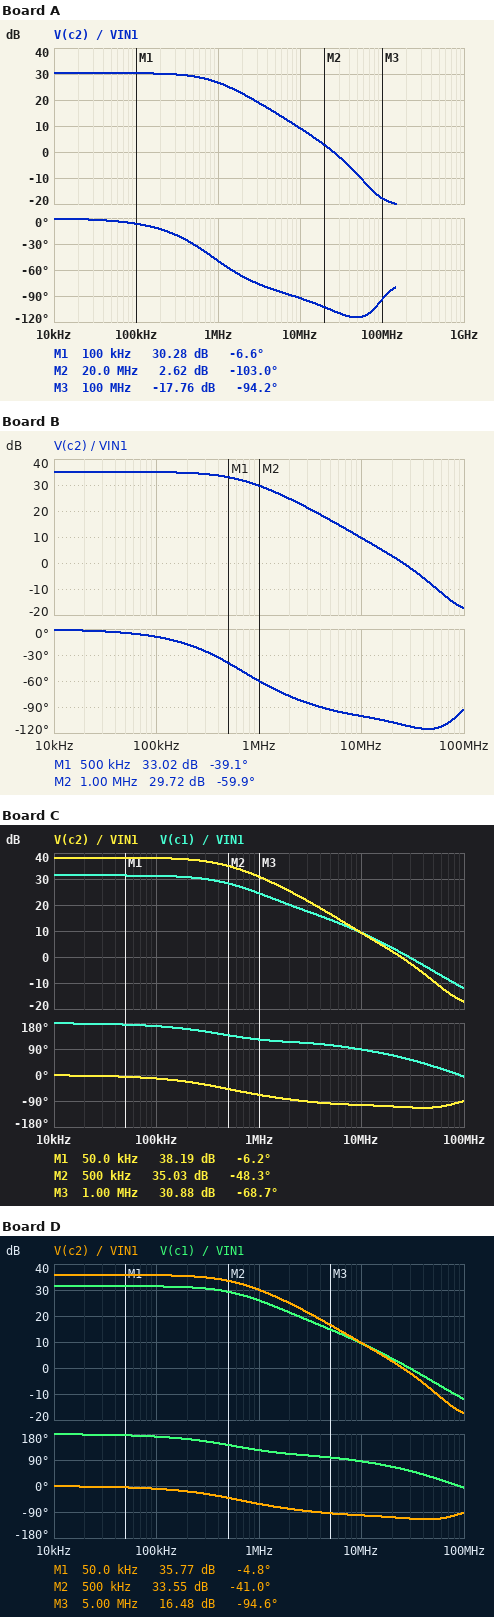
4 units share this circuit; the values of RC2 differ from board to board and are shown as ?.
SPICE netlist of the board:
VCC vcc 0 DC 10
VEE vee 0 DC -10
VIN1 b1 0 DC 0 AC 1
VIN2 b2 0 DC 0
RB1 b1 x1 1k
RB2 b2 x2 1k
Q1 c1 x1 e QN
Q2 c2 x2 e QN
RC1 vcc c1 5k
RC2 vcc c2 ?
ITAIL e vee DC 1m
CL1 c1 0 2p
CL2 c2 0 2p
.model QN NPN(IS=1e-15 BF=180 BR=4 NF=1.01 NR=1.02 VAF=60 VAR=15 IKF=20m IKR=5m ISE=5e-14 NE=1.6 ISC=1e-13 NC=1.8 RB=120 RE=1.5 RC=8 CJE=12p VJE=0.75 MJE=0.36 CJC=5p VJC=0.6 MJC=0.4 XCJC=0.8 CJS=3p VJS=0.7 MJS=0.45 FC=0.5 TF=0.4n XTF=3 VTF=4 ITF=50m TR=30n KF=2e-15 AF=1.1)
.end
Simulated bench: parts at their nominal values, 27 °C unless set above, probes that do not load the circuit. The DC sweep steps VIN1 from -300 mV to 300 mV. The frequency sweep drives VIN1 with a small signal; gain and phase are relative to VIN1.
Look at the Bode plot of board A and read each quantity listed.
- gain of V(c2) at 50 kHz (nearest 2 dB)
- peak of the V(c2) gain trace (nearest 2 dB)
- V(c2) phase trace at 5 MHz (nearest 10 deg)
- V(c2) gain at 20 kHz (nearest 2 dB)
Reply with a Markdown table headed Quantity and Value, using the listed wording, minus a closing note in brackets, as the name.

| Quantity | Value |
|---|---|
| gain of V(c2) at 50 kHz | 30 dB |
| peak of the V(c2) gain trace | 30 dB |
| V(c2) phase trace at 5 MHz | -80 deg |
| V(c2) gain at 20 kHz | 30 dB |
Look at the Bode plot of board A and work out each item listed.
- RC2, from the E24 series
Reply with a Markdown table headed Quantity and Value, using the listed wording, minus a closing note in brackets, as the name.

| Quantity | Value |
|---|---|
| RC2, from the E24 series | 4.3 kΩ |
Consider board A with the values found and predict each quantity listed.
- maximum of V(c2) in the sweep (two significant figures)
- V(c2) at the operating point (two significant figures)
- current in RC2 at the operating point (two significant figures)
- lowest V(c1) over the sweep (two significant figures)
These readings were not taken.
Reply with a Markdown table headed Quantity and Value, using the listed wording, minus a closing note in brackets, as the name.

| Quantity | Value |
|---|---|
| maximum of V(c2) in the sweep | 10 V |
| V(c2) at the operating point | 7.9 V |
| current in RC2 at the operating point | 500 µA |
| lowest V(c1) over the sweep | 5.0 V |
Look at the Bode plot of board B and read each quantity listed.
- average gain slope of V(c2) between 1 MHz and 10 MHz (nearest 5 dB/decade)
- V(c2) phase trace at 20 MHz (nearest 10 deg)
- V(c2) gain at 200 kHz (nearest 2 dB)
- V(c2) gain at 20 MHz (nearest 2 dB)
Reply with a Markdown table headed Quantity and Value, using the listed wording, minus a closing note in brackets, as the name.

| Quantity | Value |
|---|---|
| average gain slope of V(c2) between 1 MHz and 10 MHz | -20 dB/decade |
| V(c2) phase trace at 20 MHz | -110 deg |
| V(c2) gain at 200 kHz | 34 dB |
| V(c2) gain at 20 MHz | 2 dB |
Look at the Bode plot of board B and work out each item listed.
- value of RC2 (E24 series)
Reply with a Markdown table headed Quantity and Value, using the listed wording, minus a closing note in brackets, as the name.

| Quantity | Value |
|---|---|
| value of RC2 | 7.5 kΩ |
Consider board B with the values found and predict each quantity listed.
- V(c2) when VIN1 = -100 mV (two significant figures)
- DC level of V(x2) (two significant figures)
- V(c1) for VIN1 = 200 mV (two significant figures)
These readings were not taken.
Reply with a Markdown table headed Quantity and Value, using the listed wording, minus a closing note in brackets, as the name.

| Quantity | Value |
|---|---|
| V(c2) when VIN1 = -100 mV | 2.8 V |
| DC level of V(x2) | -3.8 mV |
| V(c1) for VIN1 = 200 mV | 5.0 V |
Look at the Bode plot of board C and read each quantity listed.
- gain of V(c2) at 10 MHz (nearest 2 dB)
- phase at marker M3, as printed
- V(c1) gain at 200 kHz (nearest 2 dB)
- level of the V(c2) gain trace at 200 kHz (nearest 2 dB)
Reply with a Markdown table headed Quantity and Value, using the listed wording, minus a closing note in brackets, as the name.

| Quantity | Value |
|---|---|
| gain of V(c2) at 10 MHz | 10 dB |
| phase at marker M3, as printed | -68.7 deg |
| V(c1) gain at 200 kHz | 30 dB |
| level of the V(c2) gain trace at 200 kHz | 38 dB |
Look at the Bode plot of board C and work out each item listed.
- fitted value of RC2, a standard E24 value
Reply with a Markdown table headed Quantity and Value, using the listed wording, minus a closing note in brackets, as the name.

| Quantity | Value |
|---|---|
| fitted value of RC2, a standard E24 value | 11 kΩ |
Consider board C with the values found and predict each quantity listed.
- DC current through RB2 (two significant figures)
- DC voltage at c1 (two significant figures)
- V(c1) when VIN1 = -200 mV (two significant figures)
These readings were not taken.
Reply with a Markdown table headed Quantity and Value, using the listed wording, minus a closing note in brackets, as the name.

| Quantity | Value |
|---|---|
| DC current through RB2 | 3.9 µA |
| DC voltage at c1 | 7.5 V |
| V(c1) when VIN1 = -200 mV | 10 V |
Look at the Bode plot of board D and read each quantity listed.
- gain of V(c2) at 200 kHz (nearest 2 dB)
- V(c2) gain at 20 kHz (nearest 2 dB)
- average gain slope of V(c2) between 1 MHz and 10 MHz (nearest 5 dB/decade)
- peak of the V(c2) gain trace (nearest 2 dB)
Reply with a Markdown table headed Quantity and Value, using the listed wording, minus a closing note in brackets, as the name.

| Quantity | Value |
|---|---|
| gain of V(c2) at 200 kHz | 36 dB |
| V(c2) gain at 20 kHz | 36 dB |
| average gain slope of V(c2) between 1 MHz and 10 MHz | -20 dB/decade |
| peak of the V(c2) gain trace | 36 dB |
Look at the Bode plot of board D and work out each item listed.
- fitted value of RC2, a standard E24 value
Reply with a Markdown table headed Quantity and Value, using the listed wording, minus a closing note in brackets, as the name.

| Quantity | Value |
|---|---|
| fitted value of RC2, a standard E24 value | 8.2 kΩ |
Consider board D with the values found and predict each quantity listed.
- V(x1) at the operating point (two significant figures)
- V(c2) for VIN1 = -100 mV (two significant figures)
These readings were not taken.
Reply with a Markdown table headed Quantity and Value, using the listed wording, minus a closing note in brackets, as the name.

| Quantity | Value |
|---|---|
| V(x1) at the operating point | -3.8 mV |
| V(c2) for VIN1 = -100 mV | 2.2 V |
